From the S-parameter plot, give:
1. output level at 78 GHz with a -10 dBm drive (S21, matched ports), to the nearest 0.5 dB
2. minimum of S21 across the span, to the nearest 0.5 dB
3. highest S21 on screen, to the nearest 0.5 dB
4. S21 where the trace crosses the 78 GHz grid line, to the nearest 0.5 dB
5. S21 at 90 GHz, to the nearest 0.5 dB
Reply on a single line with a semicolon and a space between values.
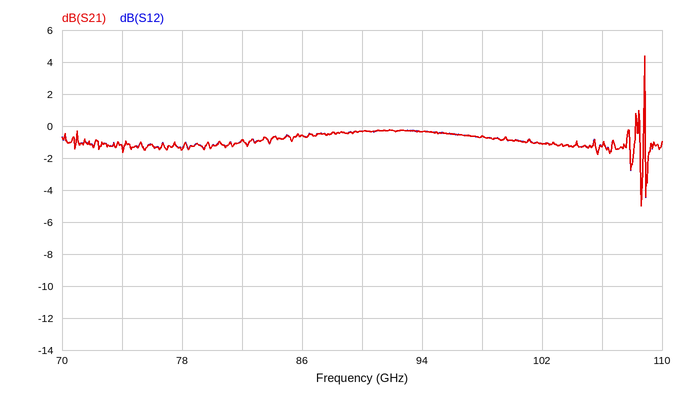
-11.5 dBm; -5.0 dB; 4.5 dB; -1.5 dB; -0.5 dB
